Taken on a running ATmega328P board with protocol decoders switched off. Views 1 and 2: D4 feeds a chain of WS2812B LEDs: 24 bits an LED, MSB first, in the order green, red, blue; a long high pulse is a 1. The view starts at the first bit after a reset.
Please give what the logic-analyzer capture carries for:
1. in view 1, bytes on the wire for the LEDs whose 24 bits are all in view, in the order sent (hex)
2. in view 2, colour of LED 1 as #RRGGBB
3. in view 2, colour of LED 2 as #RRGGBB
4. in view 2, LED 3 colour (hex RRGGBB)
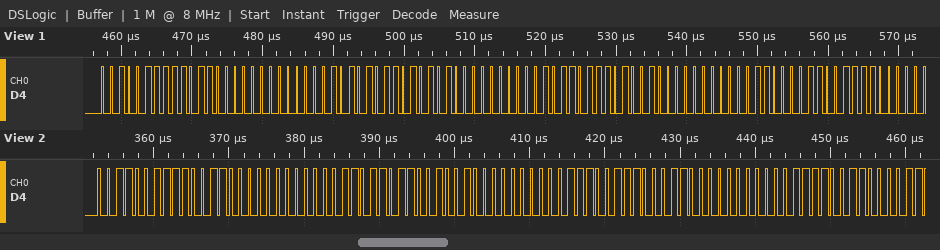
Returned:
27 D8 00 2A D5 00 2D D2 00
#CC3300
#C93600
#C63900
